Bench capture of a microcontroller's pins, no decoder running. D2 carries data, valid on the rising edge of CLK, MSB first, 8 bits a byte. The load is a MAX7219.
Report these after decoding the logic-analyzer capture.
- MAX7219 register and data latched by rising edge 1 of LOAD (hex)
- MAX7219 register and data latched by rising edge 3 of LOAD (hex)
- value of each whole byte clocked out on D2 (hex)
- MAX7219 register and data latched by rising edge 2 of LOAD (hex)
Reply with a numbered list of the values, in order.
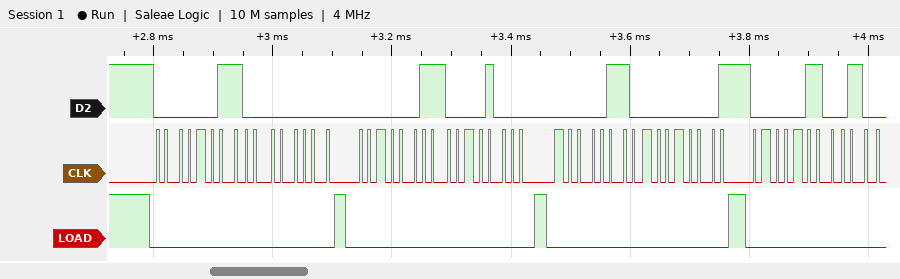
1. register 0x3, data 0x00
2. register 0x6, data 0x01
3. 03 00 03 08 06 01 06
4. register 0x3, data 0x08
